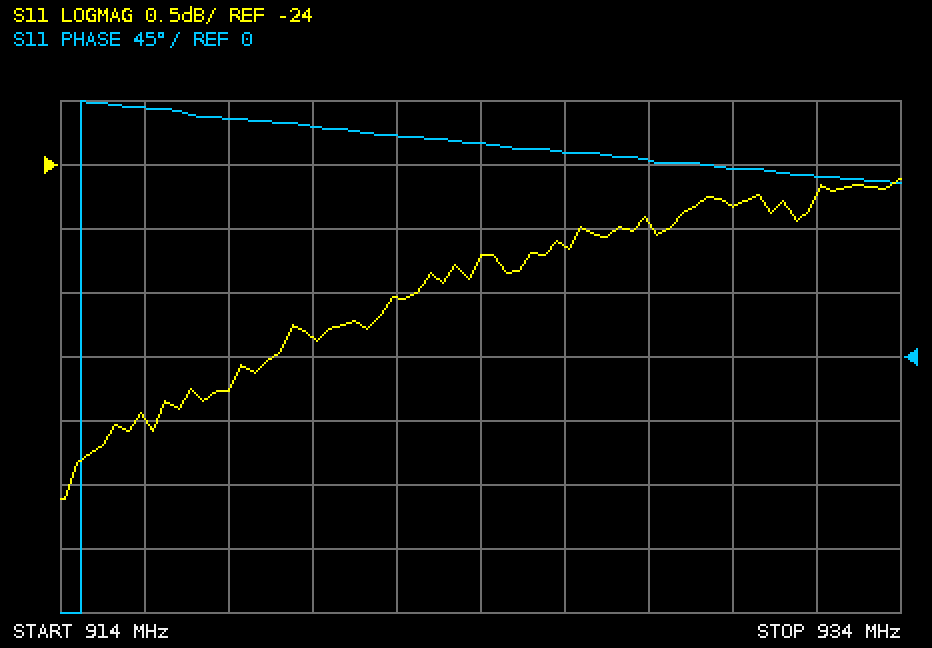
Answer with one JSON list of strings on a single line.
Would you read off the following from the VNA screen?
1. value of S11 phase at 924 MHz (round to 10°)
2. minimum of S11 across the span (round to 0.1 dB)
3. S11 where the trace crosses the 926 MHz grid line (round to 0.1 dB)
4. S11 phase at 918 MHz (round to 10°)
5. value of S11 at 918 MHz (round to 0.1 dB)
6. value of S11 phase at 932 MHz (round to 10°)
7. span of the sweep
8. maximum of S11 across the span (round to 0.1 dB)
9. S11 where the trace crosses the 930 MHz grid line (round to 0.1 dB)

["150°", "-26.6 dB", "-24.6 dB", "170°", "-25.8 dB", "130°", "20 MHz", "-24.1 dB", "-24.3 dB"]
